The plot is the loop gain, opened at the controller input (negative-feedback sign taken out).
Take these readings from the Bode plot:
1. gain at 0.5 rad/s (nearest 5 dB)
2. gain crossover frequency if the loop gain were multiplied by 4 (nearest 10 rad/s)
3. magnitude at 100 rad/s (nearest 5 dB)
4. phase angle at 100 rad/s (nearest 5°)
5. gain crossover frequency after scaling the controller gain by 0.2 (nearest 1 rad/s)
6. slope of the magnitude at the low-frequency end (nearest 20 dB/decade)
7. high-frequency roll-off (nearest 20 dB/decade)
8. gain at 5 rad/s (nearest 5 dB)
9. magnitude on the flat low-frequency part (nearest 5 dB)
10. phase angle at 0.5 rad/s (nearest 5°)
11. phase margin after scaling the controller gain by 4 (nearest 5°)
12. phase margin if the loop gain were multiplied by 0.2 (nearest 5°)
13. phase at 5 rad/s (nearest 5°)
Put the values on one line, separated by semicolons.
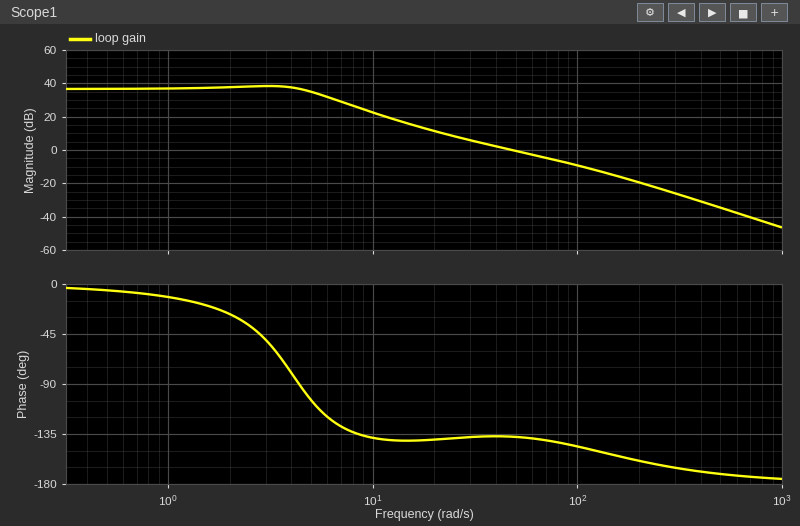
35 dB; 120 rad/s; -10 dB; -145°; 17 rad/s; 0 dB/decade; -40 dB/decade; 35 dB; 35 dB; -5°; 30°; 40°; -105°
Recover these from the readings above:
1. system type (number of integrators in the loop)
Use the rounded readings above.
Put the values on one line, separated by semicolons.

0
